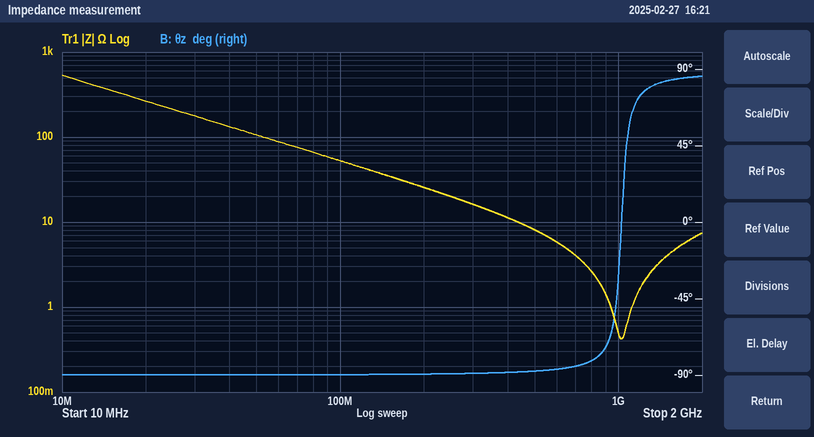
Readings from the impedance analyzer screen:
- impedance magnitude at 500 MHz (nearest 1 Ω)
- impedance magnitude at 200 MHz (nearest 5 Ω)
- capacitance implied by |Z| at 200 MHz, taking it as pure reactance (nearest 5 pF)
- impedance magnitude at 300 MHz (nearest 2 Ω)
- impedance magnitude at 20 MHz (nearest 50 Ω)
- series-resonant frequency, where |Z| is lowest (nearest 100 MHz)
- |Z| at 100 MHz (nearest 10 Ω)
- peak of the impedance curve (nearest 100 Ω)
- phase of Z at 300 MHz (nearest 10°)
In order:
8 Ω
25 Ω
30 pF
16 Ω
250 Ω
1.0 GHz
50 Ω
500 Ω
-90°
